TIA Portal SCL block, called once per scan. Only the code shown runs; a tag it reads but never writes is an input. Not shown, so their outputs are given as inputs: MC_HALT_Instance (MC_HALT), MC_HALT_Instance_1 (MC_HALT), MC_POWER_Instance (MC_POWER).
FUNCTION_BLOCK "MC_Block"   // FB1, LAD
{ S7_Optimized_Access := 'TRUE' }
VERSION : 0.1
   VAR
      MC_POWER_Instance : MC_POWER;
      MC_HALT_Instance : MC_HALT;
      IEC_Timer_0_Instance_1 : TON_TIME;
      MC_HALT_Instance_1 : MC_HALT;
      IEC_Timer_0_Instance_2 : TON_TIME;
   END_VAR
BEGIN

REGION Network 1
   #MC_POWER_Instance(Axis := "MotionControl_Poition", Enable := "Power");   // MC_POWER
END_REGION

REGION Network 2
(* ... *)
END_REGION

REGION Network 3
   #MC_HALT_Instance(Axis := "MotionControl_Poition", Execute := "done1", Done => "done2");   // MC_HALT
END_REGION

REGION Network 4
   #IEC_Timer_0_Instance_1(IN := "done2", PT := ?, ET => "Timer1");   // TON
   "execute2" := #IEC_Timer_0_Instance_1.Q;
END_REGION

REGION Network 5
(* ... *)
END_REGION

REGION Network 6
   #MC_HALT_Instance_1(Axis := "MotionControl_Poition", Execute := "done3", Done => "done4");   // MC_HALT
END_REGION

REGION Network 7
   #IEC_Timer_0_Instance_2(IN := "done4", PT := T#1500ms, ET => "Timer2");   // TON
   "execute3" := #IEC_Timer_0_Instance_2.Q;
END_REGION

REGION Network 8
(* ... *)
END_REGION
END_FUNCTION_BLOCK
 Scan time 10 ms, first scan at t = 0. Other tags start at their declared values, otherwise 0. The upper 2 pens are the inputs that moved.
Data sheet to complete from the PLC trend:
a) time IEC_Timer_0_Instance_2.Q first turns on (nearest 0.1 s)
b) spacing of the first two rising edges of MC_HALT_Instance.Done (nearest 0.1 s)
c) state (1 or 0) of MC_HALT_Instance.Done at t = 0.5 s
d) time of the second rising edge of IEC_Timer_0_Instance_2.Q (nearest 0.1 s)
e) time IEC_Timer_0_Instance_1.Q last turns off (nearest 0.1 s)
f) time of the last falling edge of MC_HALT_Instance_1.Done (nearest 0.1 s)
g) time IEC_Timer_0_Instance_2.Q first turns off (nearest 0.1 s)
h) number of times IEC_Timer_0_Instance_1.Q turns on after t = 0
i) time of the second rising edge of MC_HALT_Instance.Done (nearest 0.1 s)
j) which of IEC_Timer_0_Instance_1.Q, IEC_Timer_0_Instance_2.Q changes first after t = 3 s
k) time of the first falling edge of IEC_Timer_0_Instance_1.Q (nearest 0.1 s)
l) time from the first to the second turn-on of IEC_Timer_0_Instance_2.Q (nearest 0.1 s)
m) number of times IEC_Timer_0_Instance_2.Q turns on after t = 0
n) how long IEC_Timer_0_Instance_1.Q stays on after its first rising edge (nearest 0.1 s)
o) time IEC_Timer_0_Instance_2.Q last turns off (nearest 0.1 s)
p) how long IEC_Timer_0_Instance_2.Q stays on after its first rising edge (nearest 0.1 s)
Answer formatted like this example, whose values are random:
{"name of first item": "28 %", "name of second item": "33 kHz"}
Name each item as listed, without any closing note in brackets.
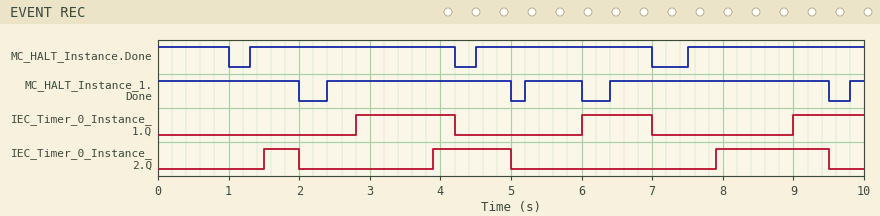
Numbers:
{"time IEC_Timer_0_Instance_2.Q first turns on": "1.5 s", "spacing of the first two rising edges of MC_HALT_Instance.Done": "3.2 s", "state (1 or 0) of MC_HALT_Instance.Done at t = 0.5 s": "1", "time of the second rising edge of IEC_Timer_0_Instance_2.Q": "3.9 s", "time IEC_Timer_0_Instance_1.Q last turns off": "7.0 s", "time of the last falling edge of MC_HALT_Instance_1.Done": "9.5 s", "time IEC_Timer_0_Instance_2.Q first turns off": "2.0 s", "number of times IEC_Timer_0_Instance_1.Q turns on after t = 0": "3", "time of the second rising edge of MC_HALT_Instance.Done": "4.5 s", "which of IEC_Timer_0_Instance_1.Q, IEC_Timer_0_Instance_2.Q changes first after t = 3 s": "IEC_Timer_0_Instance_2.Q", "time of the first falling edge of IEC_Timer_0_Instance_1.Q": "4.2 s", "time from the first to the second turn-on of IEC_Timer_0_Instance_2.Q": "2.4 s", "number of times IEC_Timer_0_Instance_2.Q turns on after t = 0": "3", "how long IEC_Timer_0_Instance_1.Q stays on after its first rising edge": "1.4 s", "time IEC_Timer_0_Instance_2.Q last turns off": "9.5 s", "how long IEC_Timer_0_Instance_2.Q stays on after its first rising edge": "0.5 s"}
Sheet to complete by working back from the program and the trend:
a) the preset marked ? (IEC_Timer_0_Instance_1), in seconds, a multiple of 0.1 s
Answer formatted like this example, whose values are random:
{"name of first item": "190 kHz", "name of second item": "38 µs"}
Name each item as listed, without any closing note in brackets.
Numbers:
{"the preset marked ? (IEC_Timer_0_Instance_1), in seconds, a multiple of 0.1 s": "1.5 s"}
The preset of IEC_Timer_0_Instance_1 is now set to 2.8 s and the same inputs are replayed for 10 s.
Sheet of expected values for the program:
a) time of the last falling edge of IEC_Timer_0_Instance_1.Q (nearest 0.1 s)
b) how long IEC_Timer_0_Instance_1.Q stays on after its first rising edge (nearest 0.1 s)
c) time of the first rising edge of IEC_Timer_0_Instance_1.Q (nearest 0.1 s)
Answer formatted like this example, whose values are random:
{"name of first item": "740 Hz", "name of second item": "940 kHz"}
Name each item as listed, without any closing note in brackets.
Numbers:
{"time of the last falling edge of IEC_Timer_0_Instance_1.Q": "4.2 s", "how long IEC_Timer_0_Instance_1.Q stays on after its first rising edge": "0.1 s", "time of the first rising edge of IEC_Timer_0_Instance_1.Q": "4.1 s"}
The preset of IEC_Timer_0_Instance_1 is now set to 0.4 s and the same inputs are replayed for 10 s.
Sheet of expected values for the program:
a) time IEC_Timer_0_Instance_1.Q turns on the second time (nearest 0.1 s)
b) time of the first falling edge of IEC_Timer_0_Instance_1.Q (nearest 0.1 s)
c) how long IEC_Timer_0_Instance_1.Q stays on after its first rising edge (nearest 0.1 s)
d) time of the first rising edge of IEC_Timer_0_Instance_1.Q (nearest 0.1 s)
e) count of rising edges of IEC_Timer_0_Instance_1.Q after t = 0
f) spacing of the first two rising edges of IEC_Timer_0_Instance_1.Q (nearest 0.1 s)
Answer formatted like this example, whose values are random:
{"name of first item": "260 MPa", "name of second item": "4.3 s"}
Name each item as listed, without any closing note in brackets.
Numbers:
{"time IEC_Timer_0_Instance_1.Q turns on the second time": "1.7 s", "time of the first falling edge of IEC_Timer_0_Instance_1.Q": "1.0 s", "how long IEC_Timer_0_Instance_1.Q stays on after its first rising edge": "0.6 s", "time of the first rising edge of IEC_Timer_0_Instance_1.Q": "0.4 s", "count of rising edges of IEC_Timer_0_Instance_1.Q after t = 0": "4", "spacing of the first two rising edges of IEC_Timer_0_Instance_1.Q": "1.3 s"}
